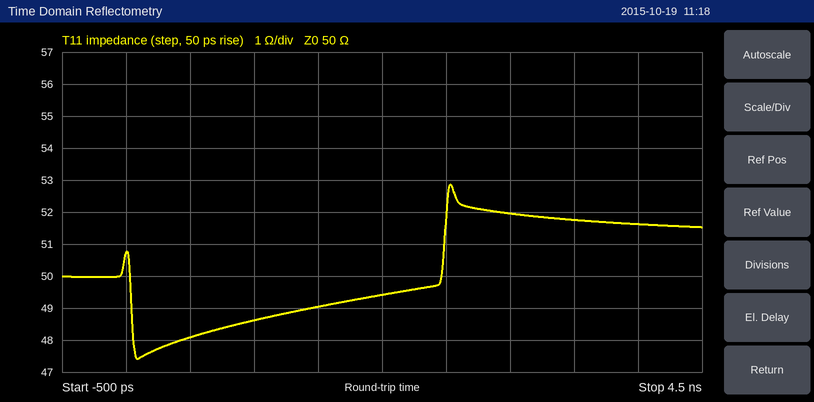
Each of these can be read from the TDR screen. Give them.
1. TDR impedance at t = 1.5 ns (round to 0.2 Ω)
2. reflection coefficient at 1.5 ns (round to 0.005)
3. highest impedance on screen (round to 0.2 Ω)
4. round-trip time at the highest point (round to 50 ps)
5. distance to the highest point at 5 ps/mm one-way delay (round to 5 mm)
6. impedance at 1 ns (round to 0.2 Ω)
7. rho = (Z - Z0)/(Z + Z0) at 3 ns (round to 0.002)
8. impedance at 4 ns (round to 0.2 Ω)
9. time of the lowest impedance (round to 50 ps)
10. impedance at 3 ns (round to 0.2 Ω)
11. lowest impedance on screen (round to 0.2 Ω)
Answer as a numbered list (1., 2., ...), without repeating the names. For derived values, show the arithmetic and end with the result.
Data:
1. 49.0 Ω
2. (49 − 50)/(49 + 50) ≈ -0.010
3. 52.8 Ω
4. 2.55 ns
5. 2.55 ns / 2 / 5 ps/mm ≈ 255 mm
6. 48.6 Ω
7. (52 − 50)/(52 + 50) ≈ +0.020
8. 51.6 Ω
9. 100 ps
10. 52.0 Ω
11. 47.4 Ω
